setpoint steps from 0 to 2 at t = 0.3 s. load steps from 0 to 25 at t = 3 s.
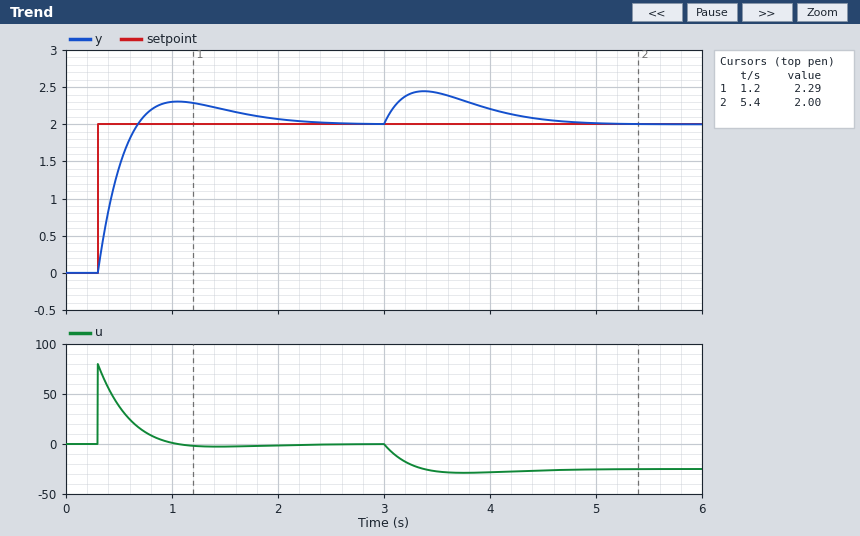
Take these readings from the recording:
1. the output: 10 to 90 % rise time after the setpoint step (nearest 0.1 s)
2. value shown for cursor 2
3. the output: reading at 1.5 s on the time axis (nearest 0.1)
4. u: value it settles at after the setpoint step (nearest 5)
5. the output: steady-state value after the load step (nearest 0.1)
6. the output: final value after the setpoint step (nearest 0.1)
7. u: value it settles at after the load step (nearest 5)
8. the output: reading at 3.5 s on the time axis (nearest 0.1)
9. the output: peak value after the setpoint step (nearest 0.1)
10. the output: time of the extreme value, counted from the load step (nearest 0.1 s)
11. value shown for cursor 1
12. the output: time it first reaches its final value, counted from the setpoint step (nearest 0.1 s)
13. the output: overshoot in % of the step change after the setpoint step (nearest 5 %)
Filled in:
0.3 s
2.00
2.2
0
2.0
2.0
-25
2.4
2.3
0.4 s
2.29
0.4 s
15 %
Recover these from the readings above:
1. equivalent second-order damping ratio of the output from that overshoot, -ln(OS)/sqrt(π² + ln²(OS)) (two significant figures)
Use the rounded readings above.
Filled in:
0.52
